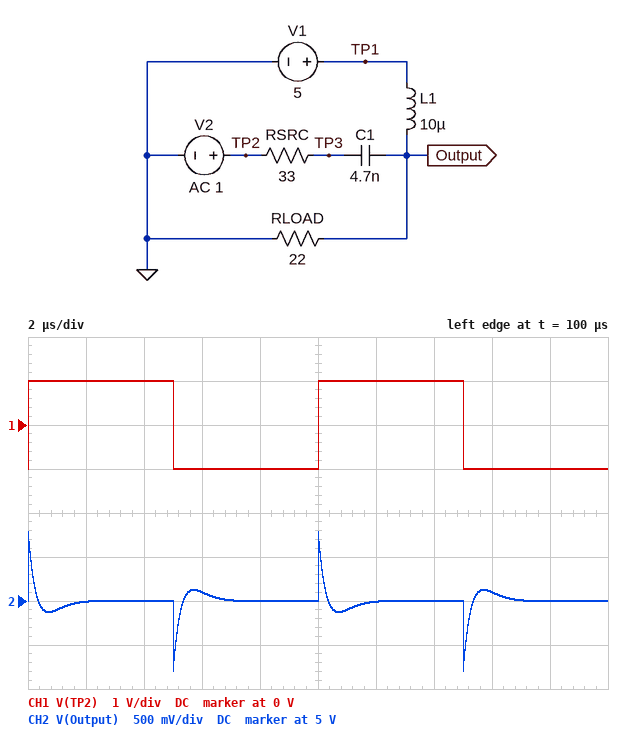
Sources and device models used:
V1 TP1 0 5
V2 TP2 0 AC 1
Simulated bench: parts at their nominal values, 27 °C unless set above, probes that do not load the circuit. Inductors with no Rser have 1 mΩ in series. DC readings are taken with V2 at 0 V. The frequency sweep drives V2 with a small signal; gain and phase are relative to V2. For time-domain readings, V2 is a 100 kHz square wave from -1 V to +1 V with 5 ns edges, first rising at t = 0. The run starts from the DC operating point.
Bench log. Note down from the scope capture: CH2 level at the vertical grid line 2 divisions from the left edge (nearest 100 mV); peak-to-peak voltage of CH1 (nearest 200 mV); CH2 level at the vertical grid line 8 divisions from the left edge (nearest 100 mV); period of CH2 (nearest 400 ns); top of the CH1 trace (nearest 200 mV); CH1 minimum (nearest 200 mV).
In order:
5.0 V
2.0 V
5.1 V
10.0 µs
1.0 V
-1.0 V
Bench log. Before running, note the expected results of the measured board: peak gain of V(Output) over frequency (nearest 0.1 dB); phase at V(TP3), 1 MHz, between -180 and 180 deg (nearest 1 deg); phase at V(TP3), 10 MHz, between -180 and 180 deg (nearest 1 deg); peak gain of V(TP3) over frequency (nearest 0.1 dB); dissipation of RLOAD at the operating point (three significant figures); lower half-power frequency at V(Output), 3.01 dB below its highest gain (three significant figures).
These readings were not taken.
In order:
-8.0 dB
-27 deg
-4 deg
0 dB
1.14 W
612 kHz
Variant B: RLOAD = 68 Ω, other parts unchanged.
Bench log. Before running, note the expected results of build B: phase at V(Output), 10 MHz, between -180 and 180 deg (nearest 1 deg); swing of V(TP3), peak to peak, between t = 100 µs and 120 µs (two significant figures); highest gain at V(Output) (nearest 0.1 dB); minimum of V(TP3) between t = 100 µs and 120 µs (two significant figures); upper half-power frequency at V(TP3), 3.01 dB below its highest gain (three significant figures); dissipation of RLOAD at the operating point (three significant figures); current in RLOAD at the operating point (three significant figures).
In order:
4 deg
2.2 V
-2.9 dB
-1.1 V
501 kHz
368 mW
73.5 mA
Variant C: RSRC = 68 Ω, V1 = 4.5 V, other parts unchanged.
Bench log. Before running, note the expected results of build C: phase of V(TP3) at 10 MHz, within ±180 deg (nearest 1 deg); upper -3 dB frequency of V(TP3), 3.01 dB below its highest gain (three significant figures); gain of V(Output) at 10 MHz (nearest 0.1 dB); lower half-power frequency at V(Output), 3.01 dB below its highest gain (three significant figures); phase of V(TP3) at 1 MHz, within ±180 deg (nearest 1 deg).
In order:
-5 deg
380 kHz
-12.2 dB
474 kHz
-37 deg
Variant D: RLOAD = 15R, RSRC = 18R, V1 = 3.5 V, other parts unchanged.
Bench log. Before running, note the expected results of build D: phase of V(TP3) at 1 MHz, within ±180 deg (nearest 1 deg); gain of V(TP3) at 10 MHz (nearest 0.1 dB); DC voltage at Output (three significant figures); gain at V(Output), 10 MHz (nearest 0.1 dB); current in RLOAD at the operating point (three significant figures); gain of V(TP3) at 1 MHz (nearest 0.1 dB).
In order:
-22 deg
-6.7 dB
3.50 V
-6.9 dB
233 mA
-2.4 dB
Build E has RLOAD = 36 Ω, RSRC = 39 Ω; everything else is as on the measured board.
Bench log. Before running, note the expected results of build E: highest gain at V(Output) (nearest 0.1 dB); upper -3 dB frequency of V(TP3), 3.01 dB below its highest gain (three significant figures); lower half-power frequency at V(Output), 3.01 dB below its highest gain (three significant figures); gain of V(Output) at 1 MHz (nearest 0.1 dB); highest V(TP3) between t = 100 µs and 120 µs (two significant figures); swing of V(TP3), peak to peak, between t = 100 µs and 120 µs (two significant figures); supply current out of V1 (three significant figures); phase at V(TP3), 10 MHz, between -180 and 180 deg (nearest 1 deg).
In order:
-6.4 dB
500 kHz
531 kHz
-6.8 dB
1.0 V
2.1 V
139 mA
-1 deg
